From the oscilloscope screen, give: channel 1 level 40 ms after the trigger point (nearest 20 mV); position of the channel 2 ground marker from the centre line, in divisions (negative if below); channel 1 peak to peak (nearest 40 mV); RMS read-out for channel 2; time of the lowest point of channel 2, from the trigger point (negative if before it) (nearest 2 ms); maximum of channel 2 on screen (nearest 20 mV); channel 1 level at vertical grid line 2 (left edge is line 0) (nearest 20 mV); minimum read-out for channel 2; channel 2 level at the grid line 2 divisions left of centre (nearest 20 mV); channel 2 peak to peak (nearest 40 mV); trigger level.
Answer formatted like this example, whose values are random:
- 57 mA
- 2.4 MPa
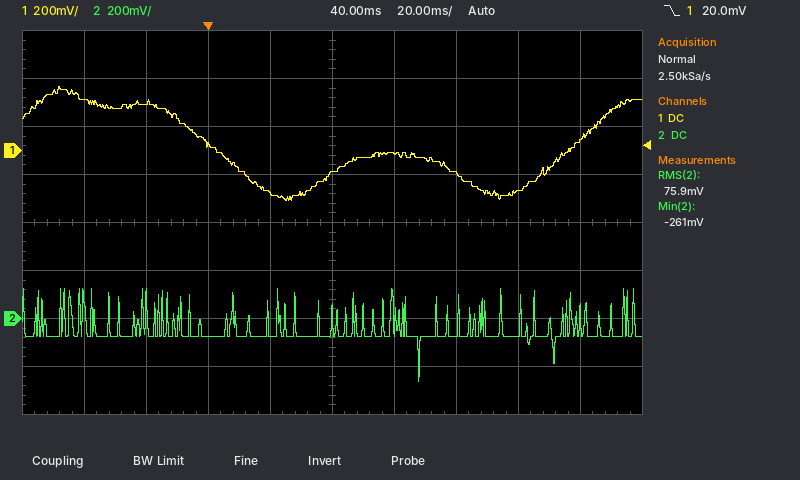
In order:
- -100 mV
- -2.0 div
- 480 mV
- 75.9 mV
- +68 ms
- 120 mV
- 200 mV
- -261 mV
- -80 mV
- 400 mV
- 20.0 mV
